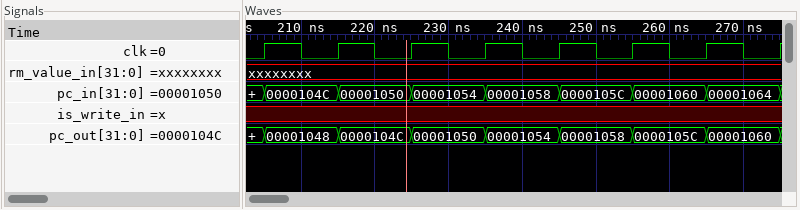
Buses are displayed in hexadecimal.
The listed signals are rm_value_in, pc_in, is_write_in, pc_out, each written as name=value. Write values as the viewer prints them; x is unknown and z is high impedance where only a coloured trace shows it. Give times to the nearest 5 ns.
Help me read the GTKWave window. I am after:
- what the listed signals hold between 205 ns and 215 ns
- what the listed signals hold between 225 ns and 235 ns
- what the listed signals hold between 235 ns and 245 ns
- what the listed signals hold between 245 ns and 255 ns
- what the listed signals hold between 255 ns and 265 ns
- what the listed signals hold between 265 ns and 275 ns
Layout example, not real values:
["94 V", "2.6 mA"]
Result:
["rm_value_in=xxxxxxxx, pc_in=0000104C, is_write_in=x, pc_out=00001048", "rm_value_in=xxxxxxxx, pc_in=00001054, is_write_in=x, pc_out=00001050", "rm_value_in=xxxxxxxx, pc_in=00001058, is_write_in=x, pc_out=00001054", "rm_value_in=xxxxxxxx, pc_in=0000105C, is_write_in=x, pc_out=00001058", "rm_value_in=xxxxxxxx, pc_in=00001060, is_write_in=x, pc_out=0000105C", "rm_value_in=xxxxxxxx, pc_in=00001064, is_write_in=x, pc_out=00001060"]
